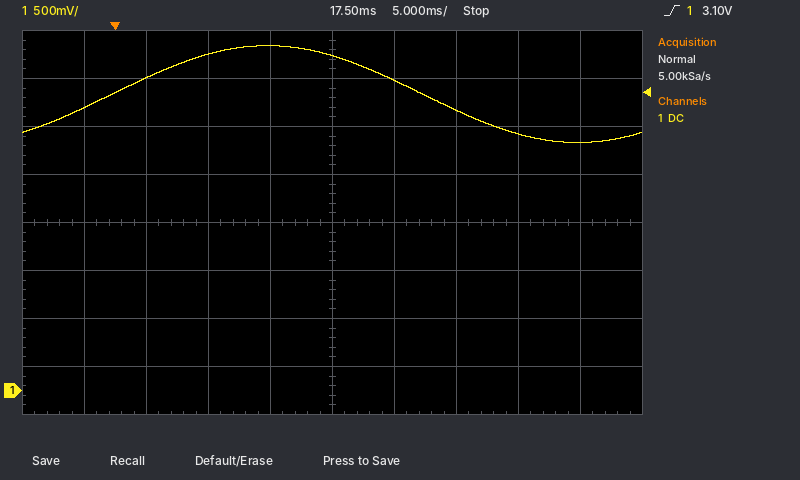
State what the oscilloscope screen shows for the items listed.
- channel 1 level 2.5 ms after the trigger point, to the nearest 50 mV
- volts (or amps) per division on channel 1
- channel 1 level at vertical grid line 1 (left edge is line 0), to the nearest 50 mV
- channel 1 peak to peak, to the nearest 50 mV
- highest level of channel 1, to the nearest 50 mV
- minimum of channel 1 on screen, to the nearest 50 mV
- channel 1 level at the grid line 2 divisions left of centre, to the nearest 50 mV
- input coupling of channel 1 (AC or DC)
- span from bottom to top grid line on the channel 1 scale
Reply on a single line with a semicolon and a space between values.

3.25 V; 500 mV; 2.95 V; 1.00 V; 3.60 V; 2.60 V; 3.50 V; DC; 4 V
